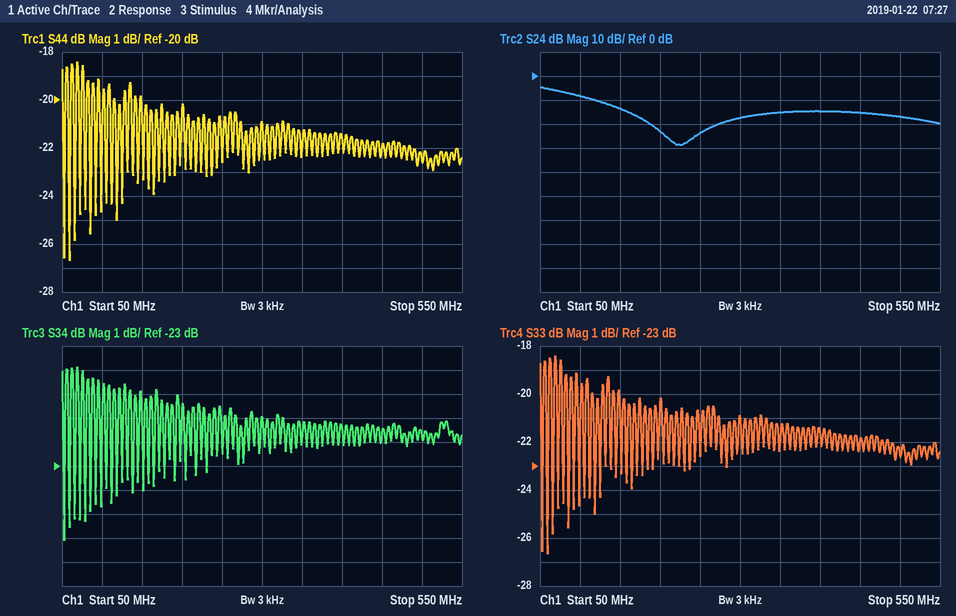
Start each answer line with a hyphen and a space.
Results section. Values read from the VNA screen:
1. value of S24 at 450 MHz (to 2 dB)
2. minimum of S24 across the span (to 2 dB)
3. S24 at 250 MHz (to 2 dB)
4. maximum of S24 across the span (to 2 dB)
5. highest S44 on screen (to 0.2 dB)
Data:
- -16 dB
- -28 dB
- -24 dB
- -4 dB
- -18.4 dB
